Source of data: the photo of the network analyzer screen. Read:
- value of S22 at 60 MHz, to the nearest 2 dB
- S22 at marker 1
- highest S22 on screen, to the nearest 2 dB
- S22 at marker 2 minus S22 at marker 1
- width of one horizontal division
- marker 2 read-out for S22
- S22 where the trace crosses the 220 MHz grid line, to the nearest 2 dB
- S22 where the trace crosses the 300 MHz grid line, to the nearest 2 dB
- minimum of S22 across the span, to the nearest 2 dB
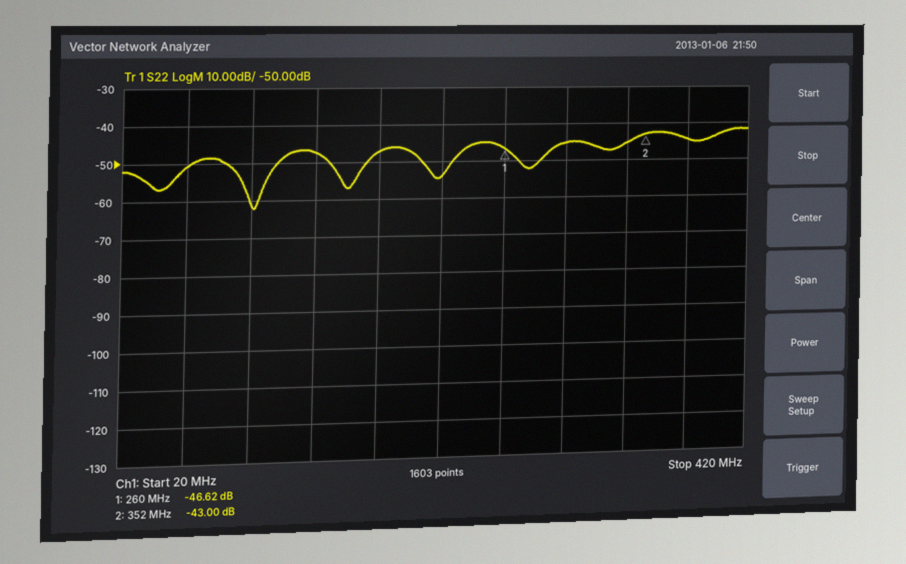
-50 dB
-46.62 dB
-42 dB
3.62 dB
40 MHz
-43.00 dB
-54 dB
-46 dB
-62 dB
